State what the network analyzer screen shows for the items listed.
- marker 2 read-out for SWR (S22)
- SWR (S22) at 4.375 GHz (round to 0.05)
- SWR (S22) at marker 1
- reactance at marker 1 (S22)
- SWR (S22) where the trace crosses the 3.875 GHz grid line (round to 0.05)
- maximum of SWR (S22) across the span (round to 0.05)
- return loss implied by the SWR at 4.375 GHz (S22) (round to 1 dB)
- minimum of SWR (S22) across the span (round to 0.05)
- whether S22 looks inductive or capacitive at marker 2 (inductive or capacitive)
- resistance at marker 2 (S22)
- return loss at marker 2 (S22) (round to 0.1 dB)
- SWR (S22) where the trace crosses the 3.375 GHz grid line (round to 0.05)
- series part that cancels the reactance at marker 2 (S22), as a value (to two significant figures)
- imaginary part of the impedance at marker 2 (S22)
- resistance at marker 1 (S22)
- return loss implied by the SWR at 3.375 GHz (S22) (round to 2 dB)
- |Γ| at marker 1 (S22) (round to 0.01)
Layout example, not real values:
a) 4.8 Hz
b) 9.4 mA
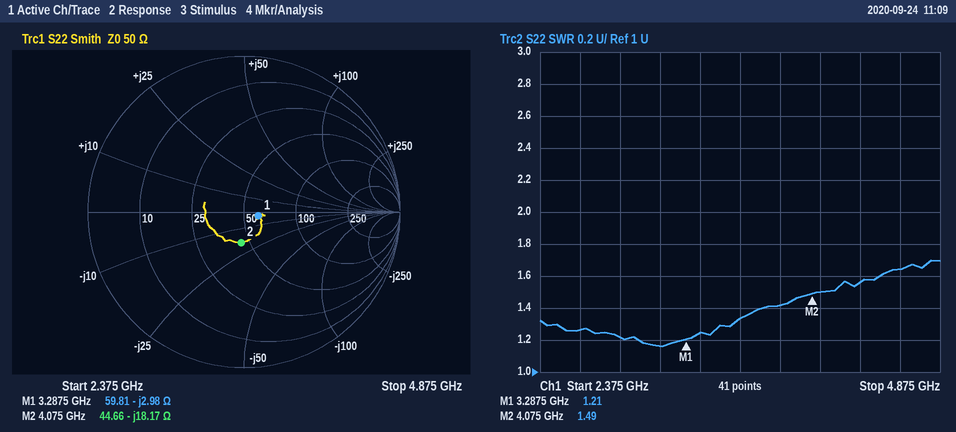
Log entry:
a) 1.49
b) 1.55
c) 1.21
d) -2.98 Ω
e) 1.40
f) 1.70
g) 13 dB
h) 1.15
i) capacitive
j) 44.66 Ω
k) 14.1 dB
l) 1.25
m) 710 pH
n) -18.17 Ω
o) 59.81 Ω
p) 20 dB
q) 0.09
